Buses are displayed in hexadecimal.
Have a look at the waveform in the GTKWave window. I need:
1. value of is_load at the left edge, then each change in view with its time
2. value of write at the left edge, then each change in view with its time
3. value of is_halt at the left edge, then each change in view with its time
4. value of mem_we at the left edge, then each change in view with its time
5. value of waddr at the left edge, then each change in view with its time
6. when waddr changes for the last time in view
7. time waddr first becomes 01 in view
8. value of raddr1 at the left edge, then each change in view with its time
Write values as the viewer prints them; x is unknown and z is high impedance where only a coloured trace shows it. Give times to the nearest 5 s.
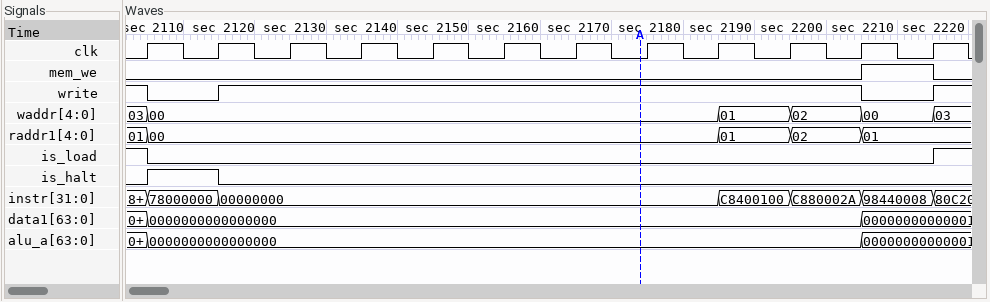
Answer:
1, 0 at 2105 s, 1 at 2215 s
1, 0 at 2105 s, 1 at 2115 s, 0 at 2205 s, 1 at 2215 s
0, 1 at 2105 s, 0 at 2115 s
0, 1 at 2205 s, 0 at 2215 s
03, 00 at 2105 s, 01 at 2185 s, 02 at 2195 s, 00 at 2205 s, 03 at 2215 s
2215 s
2185 s
01, 00 at 2105 s, 01 at 2185 s, 02 at 2195 s, 01 at 2205 s
